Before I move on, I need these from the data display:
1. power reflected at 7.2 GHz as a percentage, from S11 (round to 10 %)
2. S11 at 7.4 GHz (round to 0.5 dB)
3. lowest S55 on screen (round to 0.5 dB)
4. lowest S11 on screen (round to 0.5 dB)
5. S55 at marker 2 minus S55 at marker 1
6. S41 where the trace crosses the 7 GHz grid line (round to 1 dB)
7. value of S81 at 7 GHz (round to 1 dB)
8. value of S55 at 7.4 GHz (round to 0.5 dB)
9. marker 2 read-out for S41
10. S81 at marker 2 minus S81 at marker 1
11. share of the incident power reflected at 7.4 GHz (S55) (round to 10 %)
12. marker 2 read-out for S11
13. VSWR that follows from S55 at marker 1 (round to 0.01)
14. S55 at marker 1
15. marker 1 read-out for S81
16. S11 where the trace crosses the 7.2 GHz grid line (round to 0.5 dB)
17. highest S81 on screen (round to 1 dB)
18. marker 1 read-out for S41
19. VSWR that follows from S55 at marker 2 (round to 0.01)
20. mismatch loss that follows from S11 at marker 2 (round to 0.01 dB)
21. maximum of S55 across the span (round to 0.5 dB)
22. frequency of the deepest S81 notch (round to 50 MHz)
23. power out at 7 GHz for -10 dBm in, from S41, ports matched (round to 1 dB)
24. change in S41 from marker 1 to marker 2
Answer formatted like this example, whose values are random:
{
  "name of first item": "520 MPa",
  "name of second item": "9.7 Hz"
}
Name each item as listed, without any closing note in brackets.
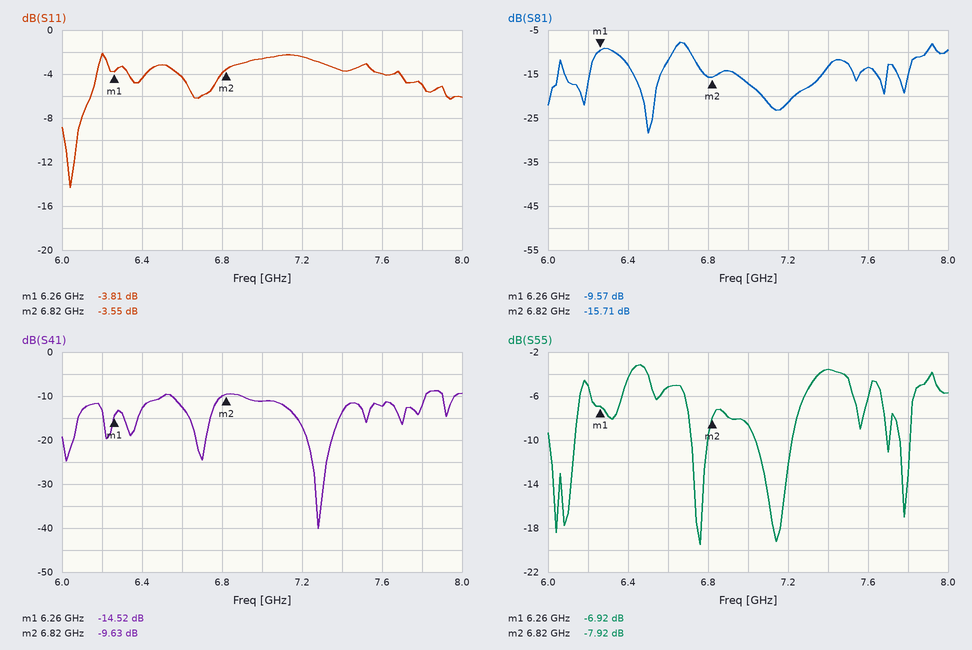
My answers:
{
  "power reflected at 7.2 GHz as a percentage, from S11": "60 %",
  "S11 at 7.4 GHz": "-3.5 dB",
  "lowest S55 on screen": "-19.5 dB",
  "lowest S11 on screen": "-14.5 dB",
  "S55 at marker 2 minus S55 at marker 1": "-1.00 dB",
  "S41 where the trace crosses the 7 GHz grid line": "-11 dB",
  "value of S81 at 7 GHz": "-17 dB",
  "value of S55 at 7.4 GHz": "-3.5 dB",
  "marker 2 read-out for S41": "-9.63 dB",
  "S81 at marker 2 minus S81 at marker 1": "-6.14 dB",
  "share of the incident power reflected at 7.4 GHz (S55)": "40 %",
  "marker 2 read-out for S11": "-3.55 dB",
  "VSWR that follows from S55 at marker 1": "2.64",
  "S55 at marker 1": "-6.92 dB",
  "marker 1 read-out for S81": "-9.57 dB",
  "S11 where the trace crosses the 7.2 GHz grid line": "-2.5 dB",
  "highest S81 on screen": "-8 dB",
  "marker 1 read-out for S41": "-14.52 dB",
  "VSWR that follows from S55 at marker 2": "2.34",
  "mismatch loss that follows from S11 at marker 2": "2.53 dB",
  "maximum of S55 across the span": "-3.0 dB",
  "frequency of the deepest S81 notch": "6.50 GHz",
  "power out at 7 GHz for -10 dBm in, from S41, ports matched": "-21 dBm",
  "change in S41 from marker 1 to marker 2": "4.89 dB"
}
